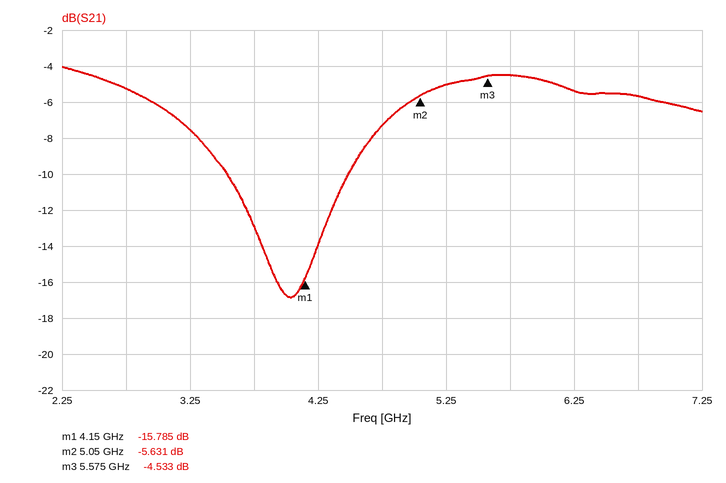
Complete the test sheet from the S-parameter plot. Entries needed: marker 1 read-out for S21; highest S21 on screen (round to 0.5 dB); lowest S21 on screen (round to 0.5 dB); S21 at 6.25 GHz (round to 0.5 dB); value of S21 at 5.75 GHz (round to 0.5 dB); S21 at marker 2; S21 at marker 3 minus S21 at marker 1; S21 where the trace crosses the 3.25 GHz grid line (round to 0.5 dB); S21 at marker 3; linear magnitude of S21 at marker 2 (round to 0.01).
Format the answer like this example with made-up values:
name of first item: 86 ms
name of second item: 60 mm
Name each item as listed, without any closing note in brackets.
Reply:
marker 1 read-out for S21: -15.785 dB
highest S21 on screen: -4.0 dB
lowest S21 on screen: -17.0 dB
S21 at 6.25 GHz: -5.5 dB
value of S21 at 5.75 GHz: -4.5 dB
S21 at marker 2: -5.631 dB
S21 at marker 3 minus S21 at marker 1: 11.252 dB
S21 where the trace crosses the 3.25 GHz grid line: -7.5 dB
S21 at marker 3: -4.533 dB
linear magnitude of S21 at marker 2: 0.52
